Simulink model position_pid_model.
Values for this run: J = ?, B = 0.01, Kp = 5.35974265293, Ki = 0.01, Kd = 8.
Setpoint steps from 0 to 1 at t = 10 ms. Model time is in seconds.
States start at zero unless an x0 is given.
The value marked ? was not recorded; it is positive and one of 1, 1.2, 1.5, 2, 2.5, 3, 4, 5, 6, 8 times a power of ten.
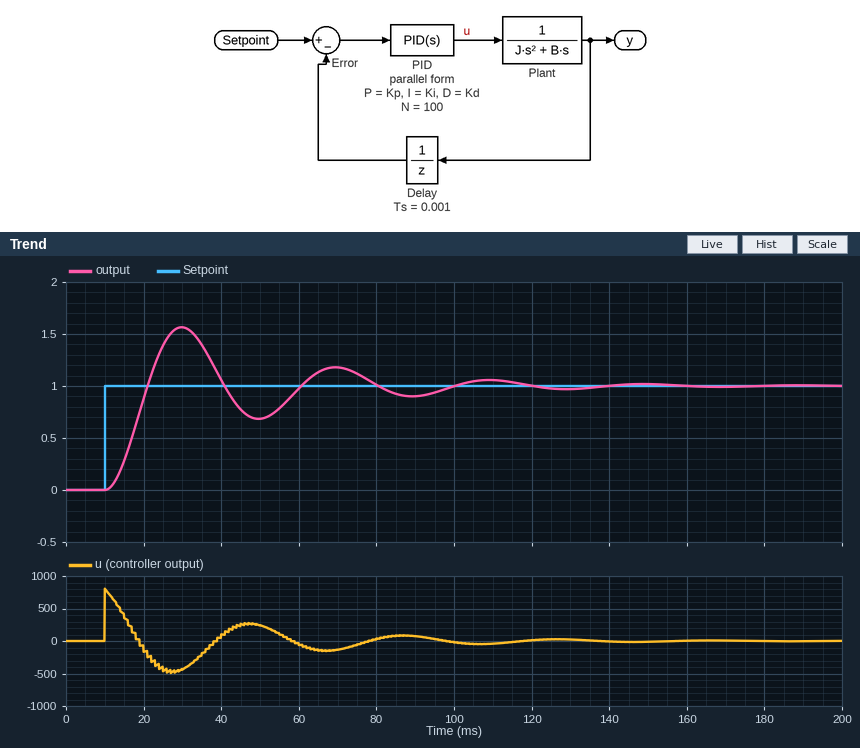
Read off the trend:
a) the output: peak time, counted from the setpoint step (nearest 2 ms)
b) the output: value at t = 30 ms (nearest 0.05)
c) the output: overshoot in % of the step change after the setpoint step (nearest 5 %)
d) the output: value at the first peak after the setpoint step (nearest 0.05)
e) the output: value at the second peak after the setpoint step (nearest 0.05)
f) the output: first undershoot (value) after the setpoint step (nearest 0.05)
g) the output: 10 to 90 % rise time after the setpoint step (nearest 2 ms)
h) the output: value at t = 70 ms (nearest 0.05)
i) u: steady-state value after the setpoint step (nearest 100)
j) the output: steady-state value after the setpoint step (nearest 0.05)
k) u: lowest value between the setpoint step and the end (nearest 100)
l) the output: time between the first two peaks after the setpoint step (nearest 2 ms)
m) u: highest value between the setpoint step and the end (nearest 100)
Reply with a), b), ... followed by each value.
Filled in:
a) 20 ms
b) 1.55
c) 55 %
d) 1.55
e) 1.20
f) 0.70
g) 8 ms
h) 1.20
i) 0
j) 1.00
k) -500
l) 40 ms
m) 800
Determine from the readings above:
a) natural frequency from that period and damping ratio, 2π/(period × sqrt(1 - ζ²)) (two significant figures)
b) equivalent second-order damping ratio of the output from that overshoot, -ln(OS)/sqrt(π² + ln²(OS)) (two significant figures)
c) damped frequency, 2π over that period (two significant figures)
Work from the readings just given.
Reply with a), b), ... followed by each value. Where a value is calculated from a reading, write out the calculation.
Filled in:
a) 2π / (40 × sqrt(1 - 0.19²)) = 0.16 rad/ms
b) ln(0.55) = -0.598; 0.598 / sqrt(9.870 + 0.357) = 0.19
c) 2π / 40 = 0.16 rad/ms
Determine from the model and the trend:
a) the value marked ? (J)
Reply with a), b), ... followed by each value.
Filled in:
a) 0.03
